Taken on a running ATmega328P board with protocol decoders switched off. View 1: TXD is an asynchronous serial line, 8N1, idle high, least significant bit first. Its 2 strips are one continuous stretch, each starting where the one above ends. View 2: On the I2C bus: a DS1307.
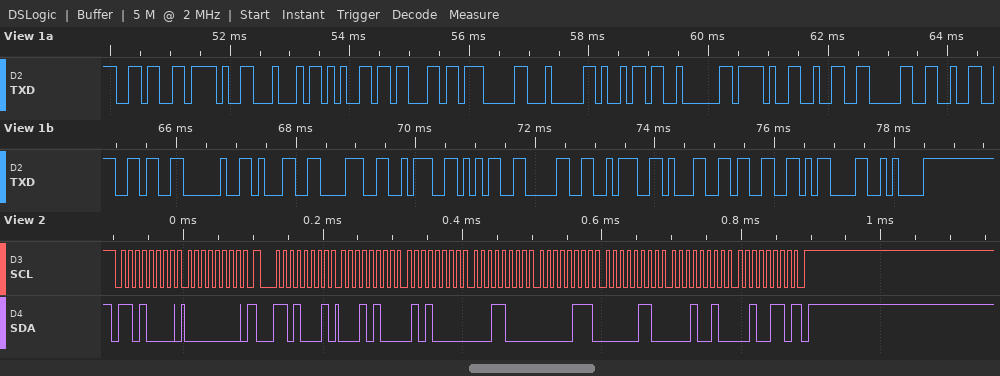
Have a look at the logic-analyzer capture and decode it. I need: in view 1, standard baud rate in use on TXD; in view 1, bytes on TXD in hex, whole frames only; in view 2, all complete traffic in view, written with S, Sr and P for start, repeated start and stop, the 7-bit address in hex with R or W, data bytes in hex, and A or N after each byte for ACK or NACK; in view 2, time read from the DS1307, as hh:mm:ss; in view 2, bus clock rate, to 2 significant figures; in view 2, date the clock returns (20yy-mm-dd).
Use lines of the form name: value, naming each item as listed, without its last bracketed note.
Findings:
in view 1, standard baud rate in use on TXD: 9600 baud
in view 1, bytes on TXD in hex, whole frames only: 36 2F 44 65 63 07 04 69 02 2F 32 30 32 36 20 31 38 3A 35 30 3A 31 33 0D 0A
in view 2, all complete traffic in view, written with S, Sr and P for start, repeated start and stop, the 7-bit address in hex with R or W, data bytes in hex, and A or N after each byte for ACK or NACK: S 68W A 00 A Sr 68R A 14 A 50 A 18 A 07 A 06 A 12 A 26 N P
in view 2, time read from the DS1307, as hh:mm:ss: 18:50:14
in view 2, bus clock rate, to 2 significant figures: 100 kHz
in view 2, date the clock returns: 2026-12-06
